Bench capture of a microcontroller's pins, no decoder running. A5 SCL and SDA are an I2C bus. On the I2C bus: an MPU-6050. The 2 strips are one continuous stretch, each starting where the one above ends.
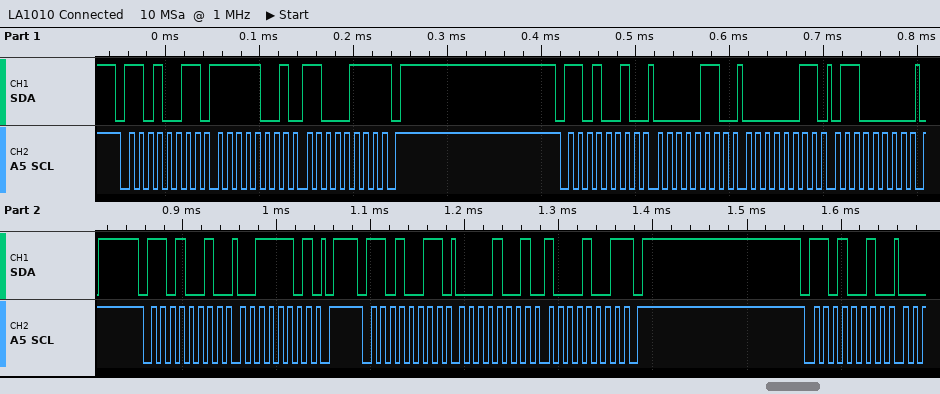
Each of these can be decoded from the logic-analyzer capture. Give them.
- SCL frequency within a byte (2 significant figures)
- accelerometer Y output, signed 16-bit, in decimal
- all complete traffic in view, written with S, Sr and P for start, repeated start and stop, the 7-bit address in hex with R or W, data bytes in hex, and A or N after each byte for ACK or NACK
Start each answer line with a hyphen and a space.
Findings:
- 100 kHz
- 2441
- S 69R A F9 A C7 N P S 69W A 06 A 03 A 60 A P S 69W A 3D A P S 69R A 09 A 89 N P S 69W A
